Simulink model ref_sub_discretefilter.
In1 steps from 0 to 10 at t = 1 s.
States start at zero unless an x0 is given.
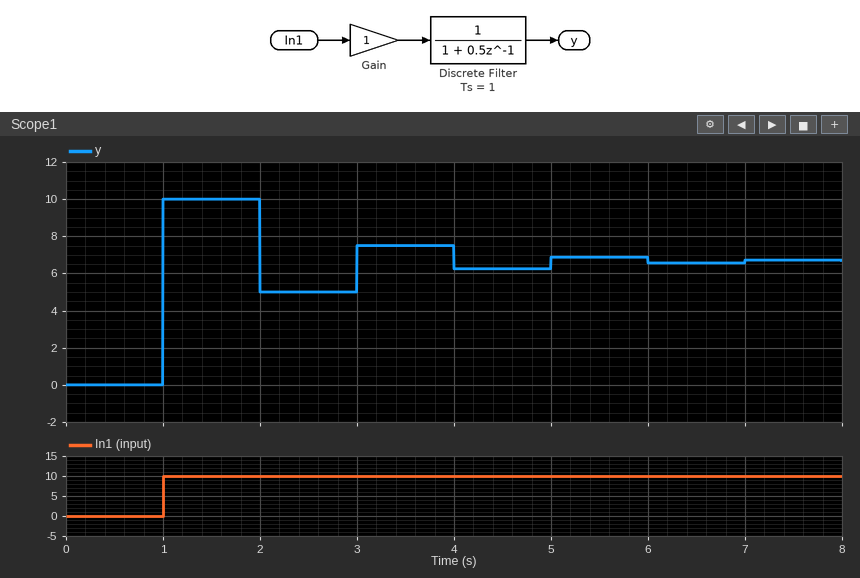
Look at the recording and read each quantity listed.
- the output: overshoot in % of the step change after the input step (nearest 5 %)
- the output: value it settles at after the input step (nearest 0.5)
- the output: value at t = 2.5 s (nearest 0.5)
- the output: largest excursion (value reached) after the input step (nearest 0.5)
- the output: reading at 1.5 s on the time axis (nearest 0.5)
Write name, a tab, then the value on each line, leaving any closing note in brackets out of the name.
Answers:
the output: overshoot in % of the step change after the input step	50 %
the output: value it settles at after the input step	6.5
the output: value at t = 2.5 s	5.0
the output: largest excursion (value reached) after the input step	10.0
the output: reading at 1.5 s on the time axis	10.0
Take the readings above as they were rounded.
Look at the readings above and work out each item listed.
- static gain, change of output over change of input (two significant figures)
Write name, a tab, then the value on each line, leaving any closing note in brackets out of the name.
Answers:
static gain, change of output over change of input	0.65
